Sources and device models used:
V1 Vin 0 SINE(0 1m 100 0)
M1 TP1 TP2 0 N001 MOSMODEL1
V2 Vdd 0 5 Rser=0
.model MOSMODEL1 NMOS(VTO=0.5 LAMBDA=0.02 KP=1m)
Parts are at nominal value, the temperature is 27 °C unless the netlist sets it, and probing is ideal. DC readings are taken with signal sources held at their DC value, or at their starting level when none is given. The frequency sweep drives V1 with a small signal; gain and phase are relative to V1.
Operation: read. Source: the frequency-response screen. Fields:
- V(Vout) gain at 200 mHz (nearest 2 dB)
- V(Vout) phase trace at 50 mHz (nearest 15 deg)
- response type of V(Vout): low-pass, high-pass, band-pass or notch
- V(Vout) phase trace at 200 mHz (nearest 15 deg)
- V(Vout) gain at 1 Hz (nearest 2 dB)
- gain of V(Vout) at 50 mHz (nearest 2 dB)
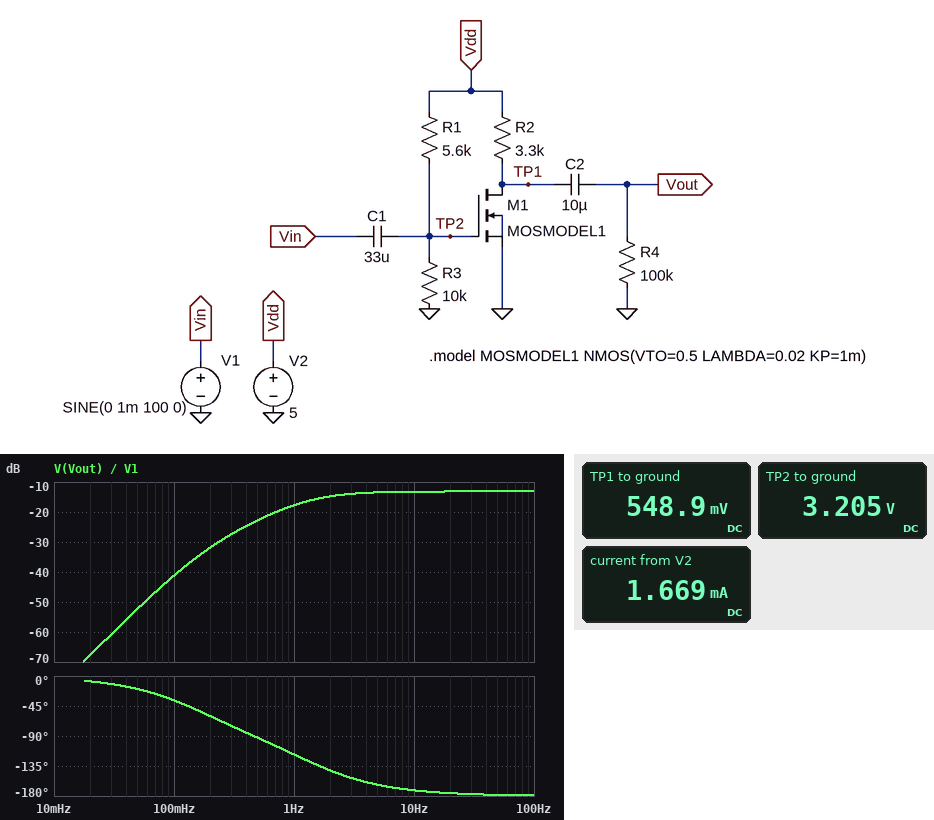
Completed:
-32 dB
-15 deg
high-pass
-60 deg
-18 dB
-52 dB
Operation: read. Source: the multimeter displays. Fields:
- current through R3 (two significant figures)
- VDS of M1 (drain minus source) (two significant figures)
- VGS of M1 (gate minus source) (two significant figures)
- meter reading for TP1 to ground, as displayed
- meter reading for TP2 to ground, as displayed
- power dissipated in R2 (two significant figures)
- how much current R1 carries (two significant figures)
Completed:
320 µA
550 mV
3.2 V
548.9 mV
3.205 V
6.0 mW
320 µA
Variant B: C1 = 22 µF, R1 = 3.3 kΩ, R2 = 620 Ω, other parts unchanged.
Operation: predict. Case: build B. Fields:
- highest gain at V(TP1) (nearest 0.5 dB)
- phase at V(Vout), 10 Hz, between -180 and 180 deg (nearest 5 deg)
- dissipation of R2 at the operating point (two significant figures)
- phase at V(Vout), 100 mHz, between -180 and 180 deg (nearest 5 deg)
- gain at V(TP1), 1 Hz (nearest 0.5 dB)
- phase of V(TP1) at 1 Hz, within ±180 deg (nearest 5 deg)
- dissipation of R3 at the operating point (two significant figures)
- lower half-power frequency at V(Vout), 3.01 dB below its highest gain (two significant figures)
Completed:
-3.0 dB
-165 deg
14 mW
-35 deg
-12.5 dB
-110 deg
1.4 mW
2.9 Hz
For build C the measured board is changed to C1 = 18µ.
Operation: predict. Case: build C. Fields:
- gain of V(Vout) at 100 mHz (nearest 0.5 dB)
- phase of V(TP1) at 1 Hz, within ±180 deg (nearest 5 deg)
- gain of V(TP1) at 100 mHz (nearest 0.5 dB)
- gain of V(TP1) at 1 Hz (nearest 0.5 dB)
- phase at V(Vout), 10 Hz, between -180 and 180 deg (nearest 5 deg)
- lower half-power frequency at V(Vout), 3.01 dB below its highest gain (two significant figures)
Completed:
-46.5 dB
-110 deg
-41.0 dB
-21.5 dB
-165 deg
2.5 Hz
